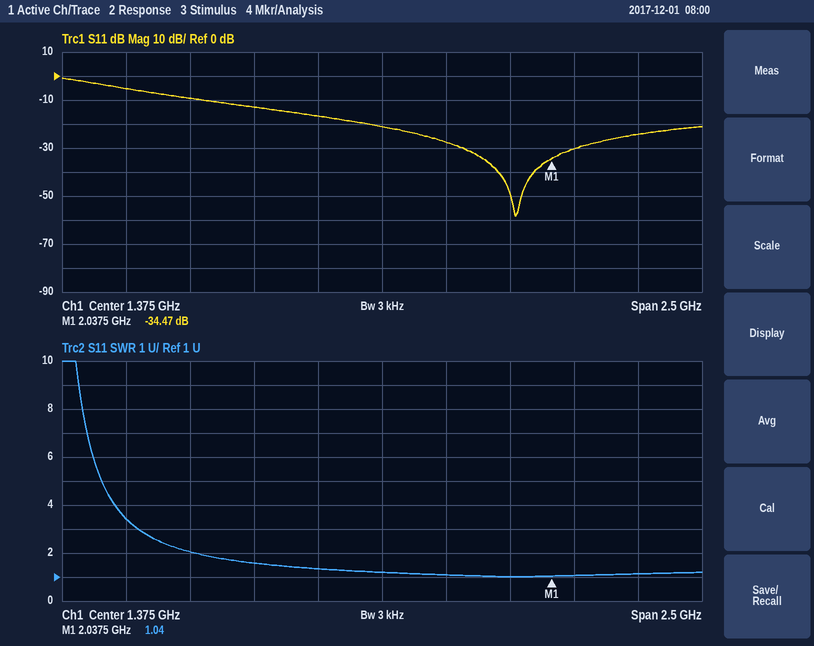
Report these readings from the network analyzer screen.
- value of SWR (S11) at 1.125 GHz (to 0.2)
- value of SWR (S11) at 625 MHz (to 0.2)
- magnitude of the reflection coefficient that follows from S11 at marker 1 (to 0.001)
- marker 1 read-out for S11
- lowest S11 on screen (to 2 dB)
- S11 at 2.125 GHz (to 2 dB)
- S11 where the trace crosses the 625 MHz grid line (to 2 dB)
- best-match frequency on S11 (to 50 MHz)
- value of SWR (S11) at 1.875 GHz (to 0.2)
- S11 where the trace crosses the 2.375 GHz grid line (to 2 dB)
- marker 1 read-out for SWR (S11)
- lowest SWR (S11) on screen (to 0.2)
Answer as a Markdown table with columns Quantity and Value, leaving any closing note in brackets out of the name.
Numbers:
| Quantity | Value |
|---|---|
| value of SWR (S11) at 1.125 GHz | 1.4 |
| value of SWR (S11) at 625 MHz | 2.0 |
| magnitude of the reflection coefficient that follows from S11 at marker 1 | 0.019 |
| marker 1 read-out for S11 | -34.47 dB |
| lowest S11 on screen | -58 dB |
| S11 at 2.125 GHz | -30 dB |
| S11 where the trace crosses the 625 MHz grid line | -10 dB |
| best-match frequency on S11 | 1.90 GHz |
| value of SWR (S11) at 1.875 GHz | 1.0 |
| S11 where the trace crosses the 2.375 GHz grid line | -24 dB |
| marker 1 read-out for SWR | 1.04 |
| lowest SWR (S11) on screen | 1.0 |
